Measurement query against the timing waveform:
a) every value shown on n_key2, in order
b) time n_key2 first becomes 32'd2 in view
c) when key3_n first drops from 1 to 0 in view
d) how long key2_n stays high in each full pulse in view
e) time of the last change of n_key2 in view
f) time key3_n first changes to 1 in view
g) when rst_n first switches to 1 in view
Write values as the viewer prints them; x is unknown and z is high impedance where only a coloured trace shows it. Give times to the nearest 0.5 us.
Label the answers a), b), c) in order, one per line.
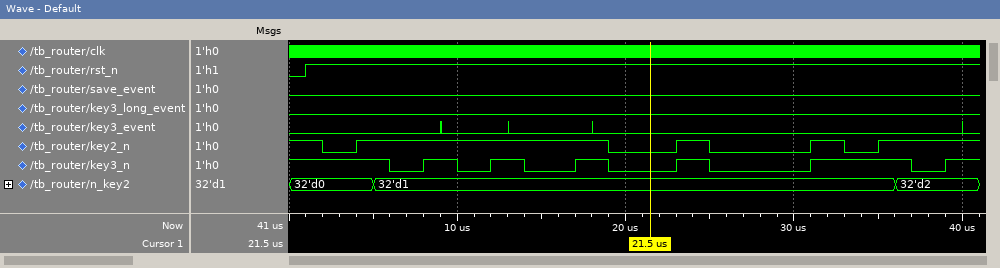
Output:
a) 32'd0, 32'd1, 32'd2
b) 36 us
c) 6 us
d) 15 us, 2 us, 2 us
e) 36 us
f) 8 us
g) 1 us
